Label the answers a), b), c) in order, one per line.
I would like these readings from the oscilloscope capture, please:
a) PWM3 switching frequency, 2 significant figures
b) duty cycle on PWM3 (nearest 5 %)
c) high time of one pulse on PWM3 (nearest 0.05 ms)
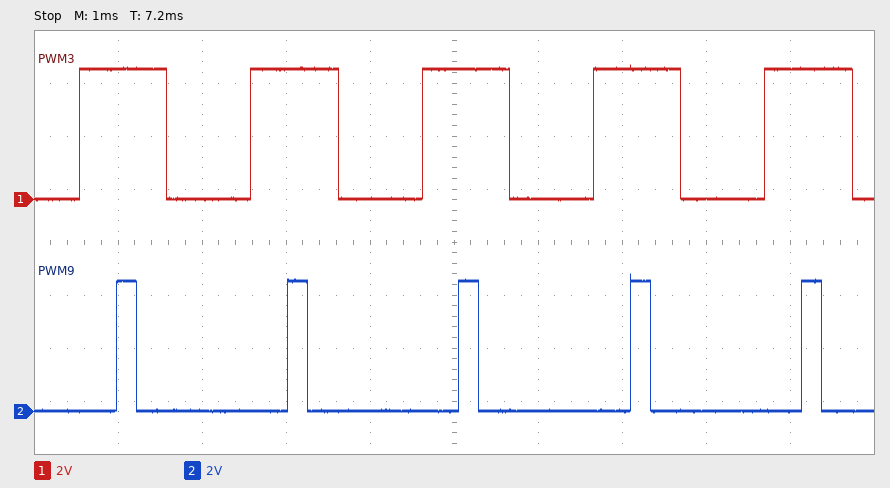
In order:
a) 490 Hz
b) 50 %
c) 1.05 ms
